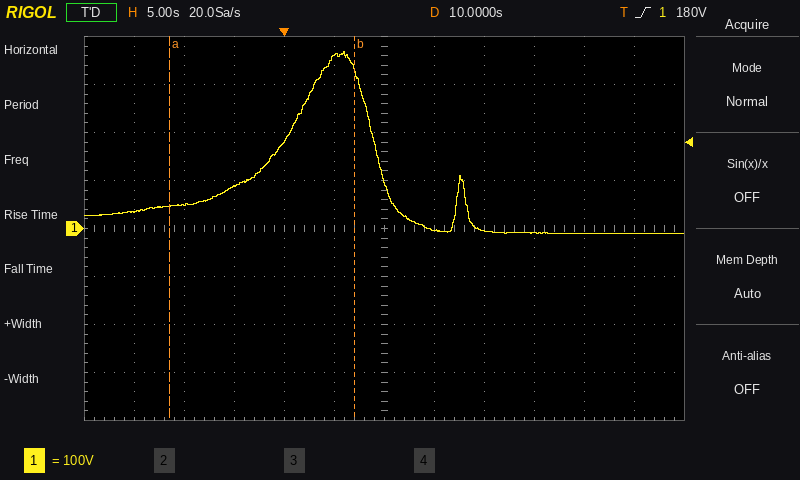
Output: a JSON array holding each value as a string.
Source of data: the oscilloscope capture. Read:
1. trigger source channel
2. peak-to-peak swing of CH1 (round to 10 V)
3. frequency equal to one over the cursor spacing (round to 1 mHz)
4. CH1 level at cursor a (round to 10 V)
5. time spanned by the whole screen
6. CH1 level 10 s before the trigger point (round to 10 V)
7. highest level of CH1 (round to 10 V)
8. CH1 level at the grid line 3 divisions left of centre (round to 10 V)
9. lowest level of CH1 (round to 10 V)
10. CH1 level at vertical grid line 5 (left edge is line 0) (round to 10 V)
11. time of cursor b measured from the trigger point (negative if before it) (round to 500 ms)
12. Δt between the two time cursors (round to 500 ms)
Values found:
["CH1", "380 V", "54 mHz", "50 V", "60 s", "50 V", "370 V", "90 V", "-10 V", "360 V", "+7.0 s", "18.5 s"]
